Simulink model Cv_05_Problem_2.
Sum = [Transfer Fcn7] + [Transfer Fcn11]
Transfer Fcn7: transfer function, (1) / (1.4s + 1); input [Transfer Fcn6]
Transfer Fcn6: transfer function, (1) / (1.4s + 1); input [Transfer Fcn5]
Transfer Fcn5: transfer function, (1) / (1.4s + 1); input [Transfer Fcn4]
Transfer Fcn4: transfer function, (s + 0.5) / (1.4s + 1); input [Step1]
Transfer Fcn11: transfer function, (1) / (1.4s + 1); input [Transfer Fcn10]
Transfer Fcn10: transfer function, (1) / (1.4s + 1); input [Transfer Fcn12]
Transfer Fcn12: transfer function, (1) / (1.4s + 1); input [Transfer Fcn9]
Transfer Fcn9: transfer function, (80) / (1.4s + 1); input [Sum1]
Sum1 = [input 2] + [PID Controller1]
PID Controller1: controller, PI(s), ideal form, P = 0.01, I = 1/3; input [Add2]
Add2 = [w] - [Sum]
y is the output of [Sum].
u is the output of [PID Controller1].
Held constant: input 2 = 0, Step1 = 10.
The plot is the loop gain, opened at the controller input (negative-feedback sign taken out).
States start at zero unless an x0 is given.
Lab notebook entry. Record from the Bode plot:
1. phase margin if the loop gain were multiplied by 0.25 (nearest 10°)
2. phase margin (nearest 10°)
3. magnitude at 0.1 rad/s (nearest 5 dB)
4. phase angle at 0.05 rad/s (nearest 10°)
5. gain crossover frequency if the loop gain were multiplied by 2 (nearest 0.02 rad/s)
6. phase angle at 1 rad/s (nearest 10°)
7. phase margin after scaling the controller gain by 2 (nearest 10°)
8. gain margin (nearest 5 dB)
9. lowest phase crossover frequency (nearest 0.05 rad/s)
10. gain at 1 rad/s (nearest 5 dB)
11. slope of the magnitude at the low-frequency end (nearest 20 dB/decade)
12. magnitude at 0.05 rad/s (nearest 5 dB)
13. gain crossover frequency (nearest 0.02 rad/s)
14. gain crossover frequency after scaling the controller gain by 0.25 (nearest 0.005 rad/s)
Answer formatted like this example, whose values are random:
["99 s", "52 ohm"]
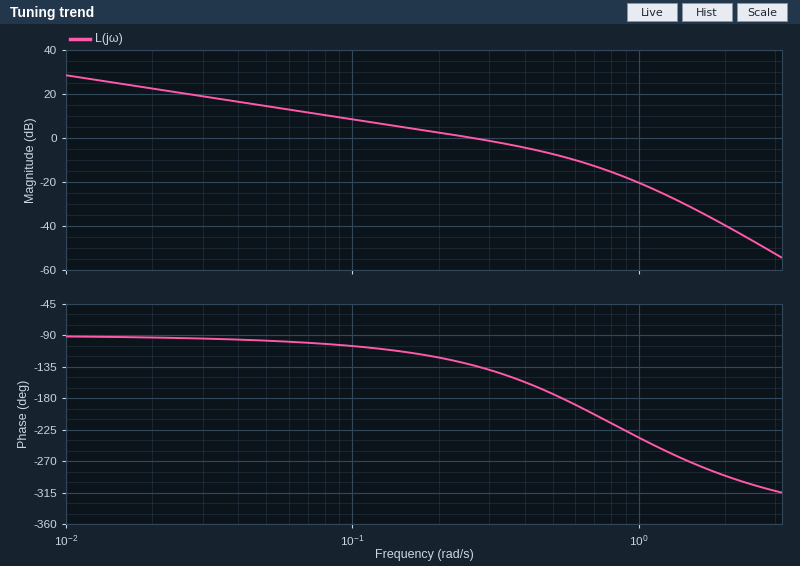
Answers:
["80°", "50°", "10 dB", "-100°", "0.46 rad/s", "-240°", "10°", "10 dB", "0.55 rad/s", "-20 dB", "-20 dB/decade", "15 dB", "0.26 rad/s", "0.065 rad/s"]
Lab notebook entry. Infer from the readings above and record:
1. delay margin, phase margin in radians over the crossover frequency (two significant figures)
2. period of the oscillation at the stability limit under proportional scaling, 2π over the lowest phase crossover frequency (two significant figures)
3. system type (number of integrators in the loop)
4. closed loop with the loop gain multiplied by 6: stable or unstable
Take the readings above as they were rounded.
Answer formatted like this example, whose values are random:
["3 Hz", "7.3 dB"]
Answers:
["3.4 s", "11 s", "1", "unstable"]
